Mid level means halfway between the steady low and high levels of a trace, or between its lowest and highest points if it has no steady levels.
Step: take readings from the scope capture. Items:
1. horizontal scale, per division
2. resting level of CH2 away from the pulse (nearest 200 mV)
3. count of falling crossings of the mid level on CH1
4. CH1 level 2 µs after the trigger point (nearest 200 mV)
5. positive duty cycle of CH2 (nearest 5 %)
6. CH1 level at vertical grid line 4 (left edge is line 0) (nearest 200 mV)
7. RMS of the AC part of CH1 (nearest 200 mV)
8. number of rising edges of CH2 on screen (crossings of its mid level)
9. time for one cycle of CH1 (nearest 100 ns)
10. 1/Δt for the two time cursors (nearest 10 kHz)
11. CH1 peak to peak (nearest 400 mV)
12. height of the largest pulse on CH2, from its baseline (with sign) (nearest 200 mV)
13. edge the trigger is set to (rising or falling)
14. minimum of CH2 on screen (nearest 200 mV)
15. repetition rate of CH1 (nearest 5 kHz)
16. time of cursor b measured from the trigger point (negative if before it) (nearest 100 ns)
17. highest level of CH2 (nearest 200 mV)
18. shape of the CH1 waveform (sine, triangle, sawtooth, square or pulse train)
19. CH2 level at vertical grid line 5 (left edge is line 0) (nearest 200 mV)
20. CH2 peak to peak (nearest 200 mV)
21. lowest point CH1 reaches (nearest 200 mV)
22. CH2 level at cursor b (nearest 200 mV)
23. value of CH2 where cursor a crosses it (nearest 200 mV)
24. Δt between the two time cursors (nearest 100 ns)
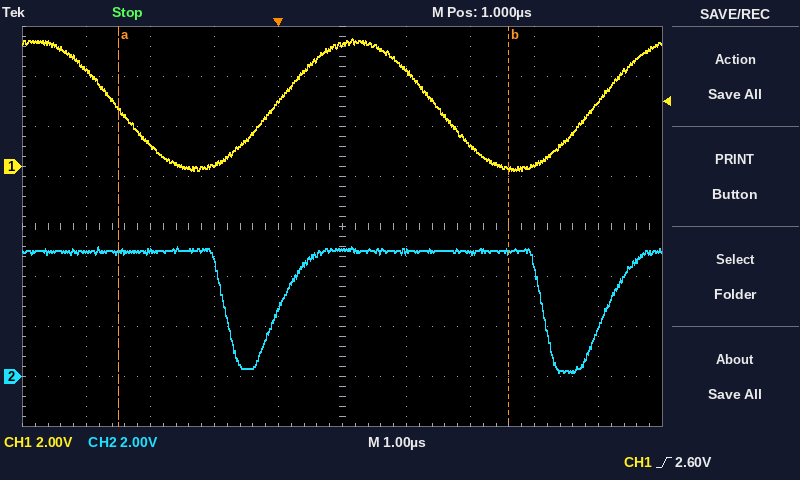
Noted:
1 µs
5.0 V
2
3.8 V
80 %
2.6 V
1.8 V
2
5.0 µs
160 kHz
5.2 V
-4.8 V
rising
200 mV
200 kHz
+3.6 µs
5.2 V
sine
5.0 V
5.0 V
-200 mV
5.0 V
5.0 V
6.1 µs
